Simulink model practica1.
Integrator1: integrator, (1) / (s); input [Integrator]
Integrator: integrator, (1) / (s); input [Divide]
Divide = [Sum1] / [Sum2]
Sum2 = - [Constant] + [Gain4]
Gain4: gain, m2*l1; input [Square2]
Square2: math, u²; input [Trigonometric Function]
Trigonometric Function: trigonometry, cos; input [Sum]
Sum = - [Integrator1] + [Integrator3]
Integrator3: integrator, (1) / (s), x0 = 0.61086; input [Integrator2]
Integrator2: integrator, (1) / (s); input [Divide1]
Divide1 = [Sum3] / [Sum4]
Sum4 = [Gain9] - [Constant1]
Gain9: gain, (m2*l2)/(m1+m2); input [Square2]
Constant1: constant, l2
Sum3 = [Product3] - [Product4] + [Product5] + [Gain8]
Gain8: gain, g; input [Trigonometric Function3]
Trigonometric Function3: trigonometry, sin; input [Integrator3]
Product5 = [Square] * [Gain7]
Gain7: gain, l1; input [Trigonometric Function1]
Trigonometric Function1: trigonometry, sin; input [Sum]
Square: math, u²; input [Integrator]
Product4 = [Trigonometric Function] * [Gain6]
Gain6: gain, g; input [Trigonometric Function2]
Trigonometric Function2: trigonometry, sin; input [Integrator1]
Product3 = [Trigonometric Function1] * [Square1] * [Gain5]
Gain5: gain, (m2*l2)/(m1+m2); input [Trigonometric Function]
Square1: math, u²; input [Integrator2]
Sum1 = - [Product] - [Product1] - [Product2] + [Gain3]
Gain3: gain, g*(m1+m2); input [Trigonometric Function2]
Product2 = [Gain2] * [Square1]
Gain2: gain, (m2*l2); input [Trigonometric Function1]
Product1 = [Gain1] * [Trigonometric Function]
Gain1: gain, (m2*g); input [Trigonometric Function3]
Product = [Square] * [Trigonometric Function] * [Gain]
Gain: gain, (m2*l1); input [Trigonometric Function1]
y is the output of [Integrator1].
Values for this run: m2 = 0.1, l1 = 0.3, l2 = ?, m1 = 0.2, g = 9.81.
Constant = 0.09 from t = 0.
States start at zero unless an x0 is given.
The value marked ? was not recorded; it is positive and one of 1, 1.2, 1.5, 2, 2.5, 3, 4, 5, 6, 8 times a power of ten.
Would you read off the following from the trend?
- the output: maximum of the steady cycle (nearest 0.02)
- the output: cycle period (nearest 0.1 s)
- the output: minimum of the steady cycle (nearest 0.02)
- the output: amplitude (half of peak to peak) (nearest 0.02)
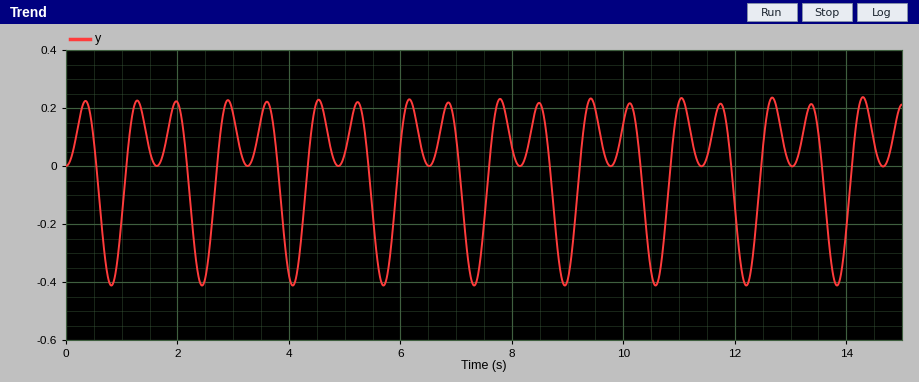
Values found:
0.24
1.6 s
-0.42
0.32
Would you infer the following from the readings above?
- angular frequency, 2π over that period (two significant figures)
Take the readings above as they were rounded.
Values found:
3.9 rad/s
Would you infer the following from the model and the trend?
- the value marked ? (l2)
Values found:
0.5
